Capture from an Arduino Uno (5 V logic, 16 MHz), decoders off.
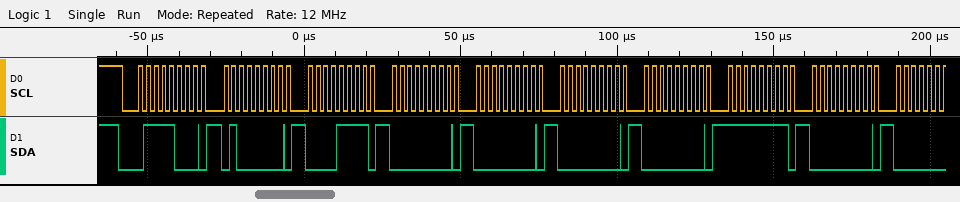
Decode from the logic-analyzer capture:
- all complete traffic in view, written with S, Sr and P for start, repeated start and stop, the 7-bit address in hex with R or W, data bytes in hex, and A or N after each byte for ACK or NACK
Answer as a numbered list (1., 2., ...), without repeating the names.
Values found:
1. S 3CW A 40 A 0F A 00 A 00 A 00 A 00 A FF A 00 A
